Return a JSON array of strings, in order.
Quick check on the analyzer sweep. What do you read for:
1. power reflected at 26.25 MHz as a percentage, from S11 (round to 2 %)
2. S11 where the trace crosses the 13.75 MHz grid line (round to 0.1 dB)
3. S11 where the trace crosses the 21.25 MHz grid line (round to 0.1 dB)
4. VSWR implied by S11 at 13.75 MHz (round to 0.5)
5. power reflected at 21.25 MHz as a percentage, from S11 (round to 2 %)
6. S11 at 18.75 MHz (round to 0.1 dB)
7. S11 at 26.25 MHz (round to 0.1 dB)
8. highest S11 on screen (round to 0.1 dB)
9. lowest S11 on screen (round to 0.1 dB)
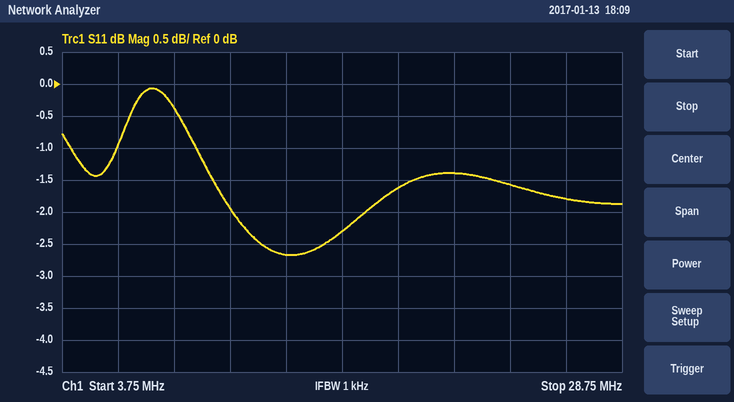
["66 %", "-2.7 dB", "-1.4 dB", "6.5", "72 %", "-1.6 dB", "-1.8 dB", "-0.1 dB", "-2.7 dB"]
